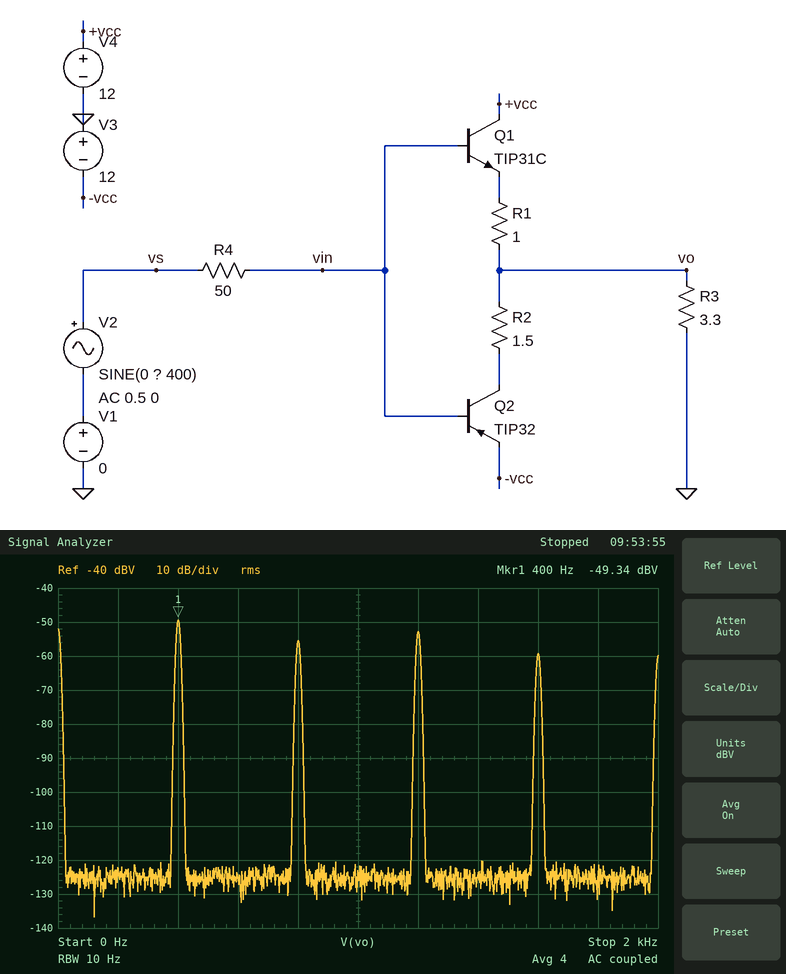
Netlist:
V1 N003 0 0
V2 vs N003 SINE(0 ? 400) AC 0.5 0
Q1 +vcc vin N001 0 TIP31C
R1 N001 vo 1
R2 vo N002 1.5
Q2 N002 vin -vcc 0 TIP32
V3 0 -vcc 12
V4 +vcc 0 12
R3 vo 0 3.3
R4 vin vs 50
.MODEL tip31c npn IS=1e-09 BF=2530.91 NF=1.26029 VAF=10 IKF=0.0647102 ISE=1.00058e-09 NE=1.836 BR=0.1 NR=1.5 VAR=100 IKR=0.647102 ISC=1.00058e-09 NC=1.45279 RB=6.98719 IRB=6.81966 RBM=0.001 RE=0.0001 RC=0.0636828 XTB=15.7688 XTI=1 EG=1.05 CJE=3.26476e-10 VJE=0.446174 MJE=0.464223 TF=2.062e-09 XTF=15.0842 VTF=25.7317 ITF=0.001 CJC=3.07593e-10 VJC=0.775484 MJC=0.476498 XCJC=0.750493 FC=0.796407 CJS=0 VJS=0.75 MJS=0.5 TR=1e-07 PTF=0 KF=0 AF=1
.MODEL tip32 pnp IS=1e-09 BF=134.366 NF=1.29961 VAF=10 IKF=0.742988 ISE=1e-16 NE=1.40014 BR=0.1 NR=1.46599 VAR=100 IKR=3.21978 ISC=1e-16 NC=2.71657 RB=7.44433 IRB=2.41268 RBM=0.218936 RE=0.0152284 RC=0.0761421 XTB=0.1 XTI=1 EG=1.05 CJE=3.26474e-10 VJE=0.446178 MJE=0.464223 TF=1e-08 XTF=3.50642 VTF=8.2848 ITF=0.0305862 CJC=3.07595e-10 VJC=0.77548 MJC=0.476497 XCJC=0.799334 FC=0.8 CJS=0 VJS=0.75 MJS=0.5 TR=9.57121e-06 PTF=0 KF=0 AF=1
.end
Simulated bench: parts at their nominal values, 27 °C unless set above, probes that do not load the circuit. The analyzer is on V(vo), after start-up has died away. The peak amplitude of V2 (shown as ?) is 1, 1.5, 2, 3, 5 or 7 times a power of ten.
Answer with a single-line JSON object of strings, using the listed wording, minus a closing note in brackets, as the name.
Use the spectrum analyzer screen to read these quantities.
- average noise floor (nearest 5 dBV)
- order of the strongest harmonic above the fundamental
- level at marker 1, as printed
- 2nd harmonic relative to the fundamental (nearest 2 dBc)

{"average noise floor": "-125 dBV", "order of the strongest harmonic above the fundamental": "3", "level at marker 1, as printed": "-49.34 dBV", "2nd harmonic relative to the fundamental": "-6 dBc"}
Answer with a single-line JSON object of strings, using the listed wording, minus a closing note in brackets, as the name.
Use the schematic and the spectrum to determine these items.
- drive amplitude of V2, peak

{"drive amplitude of V2, peak": "500 mV"}
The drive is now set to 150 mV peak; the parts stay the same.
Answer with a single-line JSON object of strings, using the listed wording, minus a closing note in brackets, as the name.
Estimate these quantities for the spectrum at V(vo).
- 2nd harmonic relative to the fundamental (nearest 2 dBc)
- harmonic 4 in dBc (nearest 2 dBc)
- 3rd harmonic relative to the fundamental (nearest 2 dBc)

{"2nd harmonic relative to the fundamental": "-14 dBc", "harmonic 4 in dBc": "-28 dBc", "3rd harmonic relative to the fundamental": "-12 dBc"}
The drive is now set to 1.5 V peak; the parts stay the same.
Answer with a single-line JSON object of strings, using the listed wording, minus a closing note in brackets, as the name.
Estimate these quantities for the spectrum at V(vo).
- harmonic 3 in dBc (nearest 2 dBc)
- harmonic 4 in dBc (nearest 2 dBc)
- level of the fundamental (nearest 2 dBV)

{"harmonic 3 in dBc": "-14 dBc", "harmonic 4 in dBc": "-34 dBc", "level of the fundamental": "-14 dBV"}
